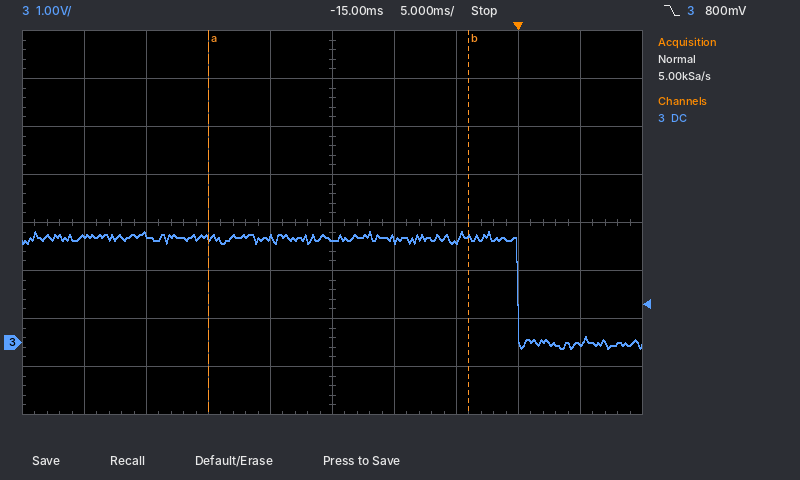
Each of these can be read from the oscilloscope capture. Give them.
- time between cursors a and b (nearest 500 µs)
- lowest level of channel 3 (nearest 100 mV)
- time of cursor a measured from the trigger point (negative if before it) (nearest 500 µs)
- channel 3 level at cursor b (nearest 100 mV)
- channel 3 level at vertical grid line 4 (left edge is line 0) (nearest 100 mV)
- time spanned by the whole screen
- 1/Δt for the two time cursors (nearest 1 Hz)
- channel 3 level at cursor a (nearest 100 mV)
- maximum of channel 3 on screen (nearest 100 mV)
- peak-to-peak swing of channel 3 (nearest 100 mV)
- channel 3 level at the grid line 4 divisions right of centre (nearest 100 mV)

21.0 ms
-100 mV
-25.0 ms
2.2 V
2.2 V
50 ms
48 Hz
2.2 V
2.3 V
2.4 V
0.0 V
